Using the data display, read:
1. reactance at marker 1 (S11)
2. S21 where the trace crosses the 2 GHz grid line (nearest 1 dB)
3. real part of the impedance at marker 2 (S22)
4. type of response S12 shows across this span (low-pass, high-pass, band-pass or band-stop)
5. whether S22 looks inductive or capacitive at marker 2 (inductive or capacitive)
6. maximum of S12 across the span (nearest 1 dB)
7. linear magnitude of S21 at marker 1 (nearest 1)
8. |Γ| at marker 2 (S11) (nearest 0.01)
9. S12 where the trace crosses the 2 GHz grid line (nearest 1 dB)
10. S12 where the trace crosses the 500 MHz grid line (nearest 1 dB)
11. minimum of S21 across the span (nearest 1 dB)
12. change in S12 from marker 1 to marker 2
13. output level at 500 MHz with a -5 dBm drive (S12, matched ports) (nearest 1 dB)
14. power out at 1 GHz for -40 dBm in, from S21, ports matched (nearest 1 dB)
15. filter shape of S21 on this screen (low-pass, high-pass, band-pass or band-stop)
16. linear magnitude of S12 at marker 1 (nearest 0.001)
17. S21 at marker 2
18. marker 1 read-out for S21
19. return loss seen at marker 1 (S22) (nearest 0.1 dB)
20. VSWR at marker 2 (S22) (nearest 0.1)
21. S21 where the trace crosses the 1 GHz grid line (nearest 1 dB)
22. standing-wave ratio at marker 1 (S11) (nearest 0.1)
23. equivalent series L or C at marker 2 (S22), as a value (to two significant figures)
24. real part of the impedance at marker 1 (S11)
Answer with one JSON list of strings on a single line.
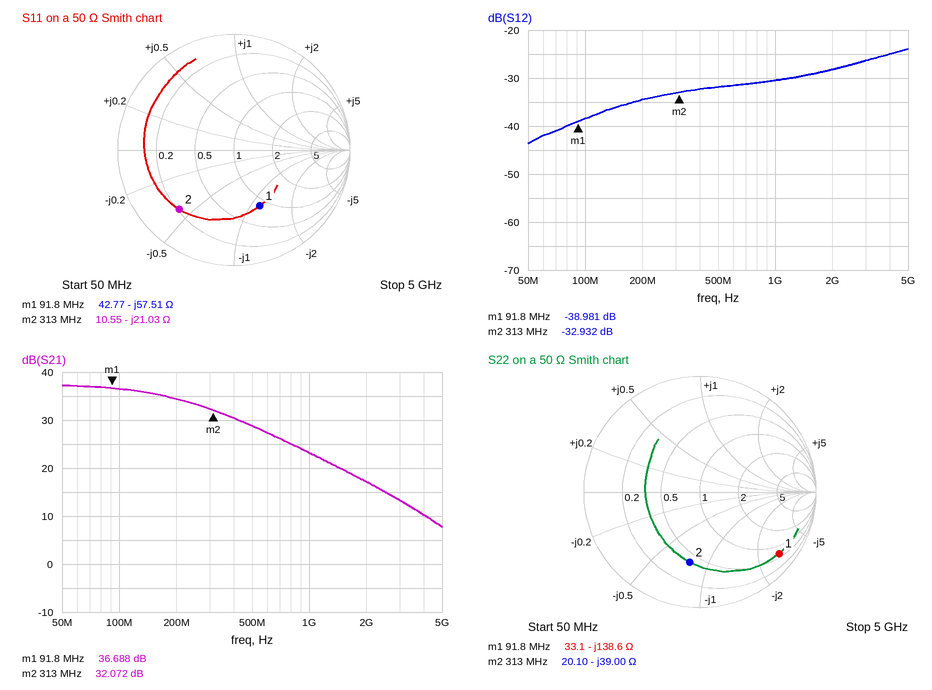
["-57.51 Ω", "17 dB", "20.10 Ω", "high-pass", "capacitive", "-24 dB", "68", "0.70", "-28 dB", "-32 dB", "8 dB", "6.049 dB", "-37 dBm", "-17 dBm", "low-pass", "0.011", "32.072 dB", "36.688 dB", "1.3 dB", "4.2", "23 dB", "3.3", "13 pF", "42.77 Ω"]
